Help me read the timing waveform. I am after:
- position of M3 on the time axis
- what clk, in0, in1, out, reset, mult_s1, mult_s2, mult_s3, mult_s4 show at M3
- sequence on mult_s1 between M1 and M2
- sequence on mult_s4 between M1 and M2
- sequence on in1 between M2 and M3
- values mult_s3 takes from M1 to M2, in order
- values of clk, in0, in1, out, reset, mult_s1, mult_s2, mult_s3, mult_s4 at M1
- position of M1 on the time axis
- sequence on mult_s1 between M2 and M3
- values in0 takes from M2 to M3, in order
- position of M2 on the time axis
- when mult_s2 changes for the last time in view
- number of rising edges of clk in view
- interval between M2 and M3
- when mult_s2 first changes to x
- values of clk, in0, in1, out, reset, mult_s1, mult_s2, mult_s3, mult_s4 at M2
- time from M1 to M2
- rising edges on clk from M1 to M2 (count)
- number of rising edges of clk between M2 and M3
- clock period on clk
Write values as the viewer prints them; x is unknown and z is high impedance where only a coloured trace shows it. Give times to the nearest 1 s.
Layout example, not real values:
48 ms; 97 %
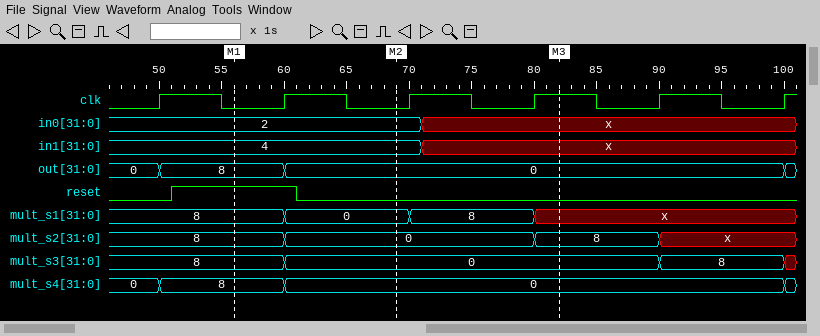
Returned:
82 s; clk=1, in0=x, in1=x, out=0, reset=0, mult_s1=x, mult_s2=8, mult_s3=0, mult_s4=0; 8, 0; 8, 0; 4, x; 8, 0; clk=0, in0=2, in1=4, out=8, reset=1, mult_s1=8, mult_s2=8, mult_s3=8, mult_s4=8; 56 s; 0, 8, x; 2, x; 69 s; 90 s; 6; 13 s; 90 s; clk=0, in0=2, in1=4, out=0, reset=0, mult_s1=0, mult_s2=0, mult_s3=0, mult_s4=0; 13 s; 1; 2; 10 s
